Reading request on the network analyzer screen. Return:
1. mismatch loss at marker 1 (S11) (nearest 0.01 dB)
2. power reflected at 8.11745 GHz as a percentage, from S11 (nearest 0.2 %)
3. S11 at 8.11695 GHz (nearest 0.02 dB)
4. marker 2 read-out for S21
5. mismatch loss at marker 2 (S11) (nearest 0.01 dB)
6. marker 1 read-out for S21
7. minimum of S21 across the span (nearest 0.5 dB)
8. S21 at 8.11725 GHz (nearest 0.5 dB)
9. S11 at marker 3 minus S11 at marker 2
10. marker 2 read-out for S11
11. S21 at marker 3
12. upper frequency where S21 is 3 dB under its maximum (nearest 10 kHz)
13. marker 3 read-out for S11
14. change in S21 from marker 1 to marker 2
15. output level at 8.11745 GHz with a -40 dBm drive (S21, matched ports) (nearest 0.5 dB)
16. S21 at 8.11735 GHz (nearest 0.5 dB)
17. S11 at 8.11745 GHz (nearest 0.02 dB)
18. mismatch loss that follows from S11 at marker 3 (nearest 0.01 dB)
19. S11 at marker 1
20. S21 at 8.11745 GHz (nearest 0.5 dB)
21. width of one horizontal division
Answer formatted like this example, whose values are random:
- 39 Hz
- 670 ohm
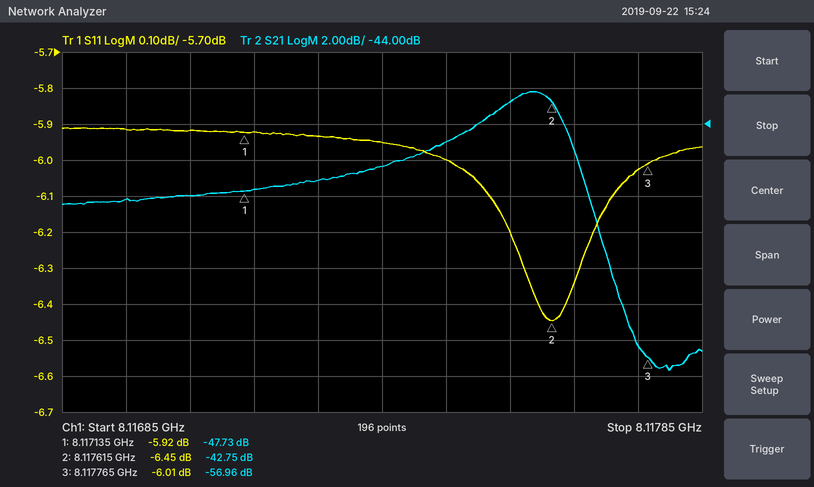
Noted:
- 1.28 dB
- 25.2 %
- -5.92 dB
- -42.75 dB
- 1.12 dB
- -47.73 dB
- -57.5 dB
- -47.0 dB
- 0.44 dB
- -6.45 dB
- -56.96 dB
- 8.11765 GHz
- -6.01 dB
- 4.98 dB
- -85.0 dBm
- -46.5 dB
- -6.00 dB
- 1.25 dB
- -5.92 dB
- -45.0 dB
- 100 kHz
